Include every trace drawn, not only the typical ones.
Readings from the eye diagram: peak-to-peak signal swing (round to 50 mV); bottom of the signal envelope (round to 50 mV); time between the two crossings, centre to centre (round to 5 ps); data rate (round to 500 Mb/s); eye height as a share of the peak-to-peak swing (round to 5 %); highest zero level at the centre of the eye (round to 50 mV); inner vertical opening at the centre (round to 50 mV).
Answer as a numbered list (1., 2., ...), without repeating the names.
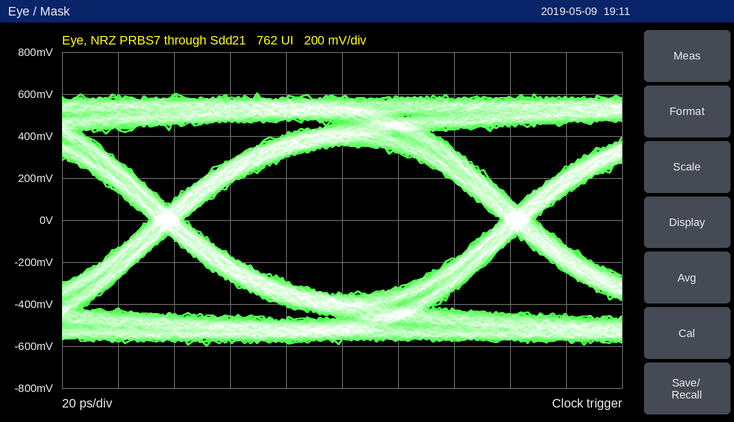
1. 1.20 V
2. -600 mV
3. 125 ps
4. 8.0 Gb/s
5. 60 %
6. -350 mV
7. 700 mV
